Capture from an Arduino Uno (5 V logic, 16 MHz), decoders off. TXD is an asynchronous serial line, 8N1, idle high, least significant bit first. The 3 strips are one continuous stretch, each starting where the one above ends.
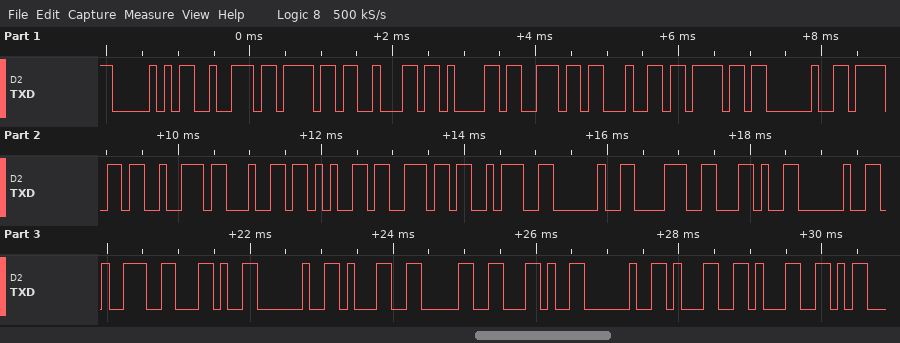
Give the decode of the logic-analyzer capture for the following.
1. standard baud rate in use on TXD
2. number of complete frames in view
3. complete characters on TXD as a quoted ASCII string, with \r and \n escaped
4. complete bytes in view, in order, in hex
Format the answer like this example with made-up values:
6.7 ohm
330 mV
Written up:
9600 baud
28
"Probando orden: 8, 9, 10, 11"
50 72 6F 62 61 6E 64 6F 20 6F 72 64 65 6E 3A 20 38 2C 20 39 2C 20 31 30 2C 20 31 31
